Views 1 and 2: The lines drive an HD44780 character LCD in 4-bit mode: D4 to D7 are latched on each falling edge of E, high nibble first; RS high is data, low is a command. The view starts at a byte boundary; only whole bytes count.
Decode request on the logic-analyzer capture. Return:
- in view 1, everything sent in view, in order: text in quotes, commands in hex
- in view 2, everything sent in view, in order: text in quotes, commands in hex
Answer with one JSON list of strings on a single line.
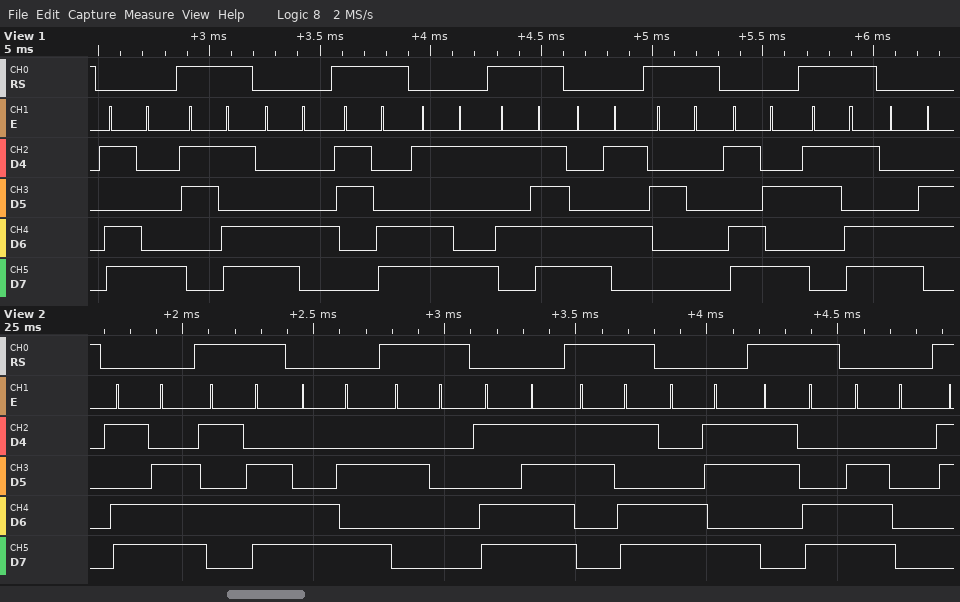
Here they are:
["0xD8 \"=\" 0xC4 \"<\" 0xD9 \"_\" 0xC5 \" \" 0xDA \"=\" 0xC6", "0xDE \"^\" 0xCA \" \" 0xDF \"=\" 0xCB \"<\" 0xE0"]
